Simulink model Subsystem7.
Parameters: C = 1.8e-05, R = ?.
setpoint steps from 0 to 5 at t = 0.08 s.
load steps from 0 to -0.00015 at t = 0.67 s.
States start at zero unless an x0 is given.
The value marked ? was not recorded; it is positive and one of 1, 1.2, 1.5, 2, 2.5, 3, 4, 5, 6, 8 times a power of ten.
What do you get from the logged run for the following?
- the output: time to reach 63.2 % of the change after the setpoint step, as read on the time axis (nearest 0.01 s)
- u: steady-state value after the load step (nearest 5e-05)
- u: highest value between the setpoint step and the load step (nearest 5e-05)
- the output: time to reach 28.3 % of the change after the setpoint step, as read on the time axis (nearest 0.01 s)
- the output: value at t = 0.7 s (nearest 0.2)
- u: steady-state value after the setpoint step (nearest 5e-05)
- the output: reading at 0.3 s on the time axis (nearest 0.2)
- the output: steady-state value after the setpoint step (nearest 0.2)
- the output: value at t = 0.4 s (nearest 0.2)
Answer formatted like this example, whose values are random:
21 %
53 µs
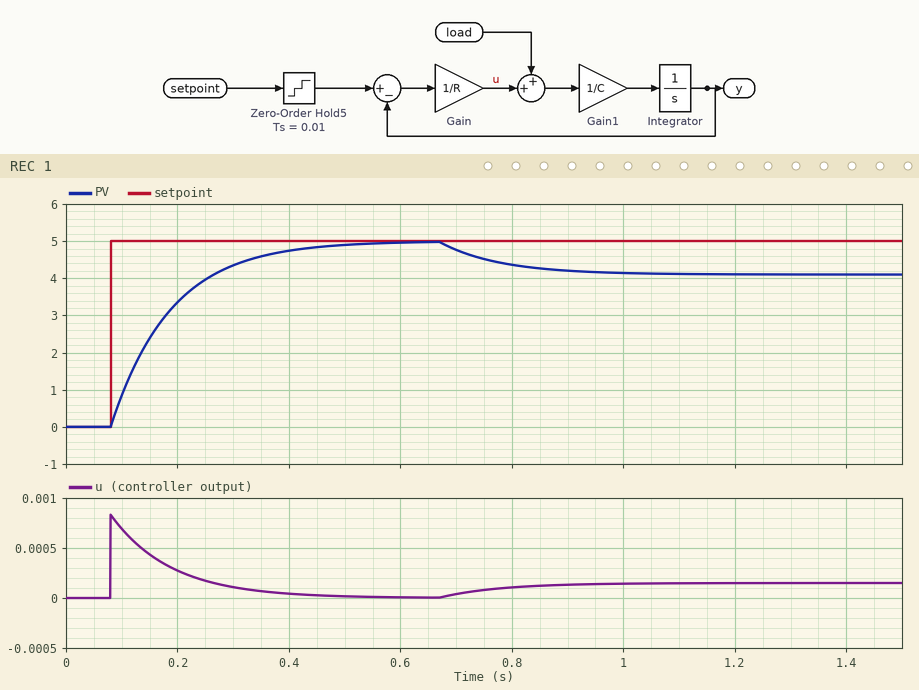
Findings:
0.19 s
0.00015
0.00085
0.12 s
4.8
0.00000
4.4
5.0
4.8
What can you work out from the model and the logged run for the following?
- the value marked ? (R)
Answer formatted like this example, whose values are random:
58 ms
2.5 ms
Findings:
6000
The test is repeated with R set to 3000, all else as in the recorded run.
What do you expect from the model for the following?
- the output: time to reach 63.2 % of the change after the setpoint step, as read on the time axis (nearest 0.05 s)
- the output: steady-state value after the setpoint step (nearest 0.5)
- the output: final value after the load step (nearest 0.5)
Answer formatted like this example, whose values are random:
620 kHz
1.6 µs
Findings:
0.15 s
5.0
4.5
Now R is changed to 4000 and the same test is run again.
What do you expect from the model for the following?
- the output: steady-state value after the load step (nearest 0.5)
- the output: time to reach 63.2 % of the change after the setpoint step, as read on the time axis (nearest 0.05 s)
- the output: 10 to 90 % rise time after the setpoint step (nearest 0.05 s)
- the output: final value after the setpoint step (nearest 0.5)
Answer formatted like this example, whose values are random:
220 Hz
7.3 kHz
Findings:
4.5
0.15 s
0.15 s
5.0
